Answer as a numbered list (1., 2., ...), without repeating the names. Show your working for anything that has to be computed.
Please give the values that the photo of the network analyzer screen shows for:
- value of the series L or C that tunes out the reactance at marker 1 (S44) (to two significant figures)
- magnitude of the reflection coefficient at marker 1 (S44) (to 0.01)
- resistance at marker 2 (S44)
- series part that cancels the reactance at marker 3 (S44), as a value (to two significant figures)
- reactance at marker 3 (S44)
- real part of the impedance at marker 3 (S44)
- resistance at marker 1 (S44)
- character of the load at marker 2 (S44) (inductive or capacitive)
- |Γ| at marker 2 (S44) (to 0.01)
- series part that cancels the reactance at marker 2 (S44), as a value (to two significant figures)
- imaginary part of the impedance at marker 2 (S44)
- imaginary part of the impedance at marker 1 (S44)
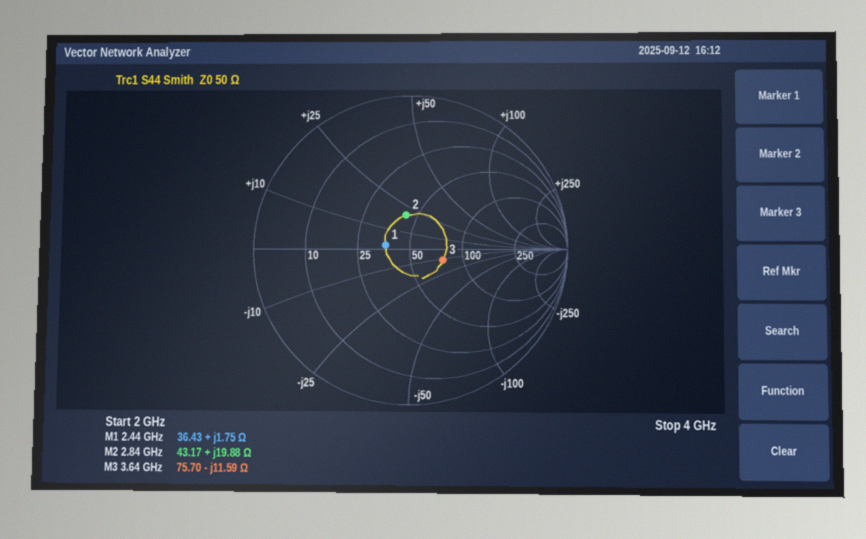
1. C = 1/(2π × 2.44 GHz × 1.75 Ω) ≈ 37 pF
2. 0.16
3. 43.17 Ω
4. L = 11.59 Ω/(2π × 3.64 GHz) ≈ 507 pH, so 510 pH to two significant figures
5. -11.59 Ω
6. 75.70 Ω
7. 36.43 Ω
8. inductive
9. 0.22
10. C = 1/(2π × 2.84 GHz × 19.88 Ω) ≈ 2.8 pF
11. +19.88 Ω
12. +1.75 Ω
